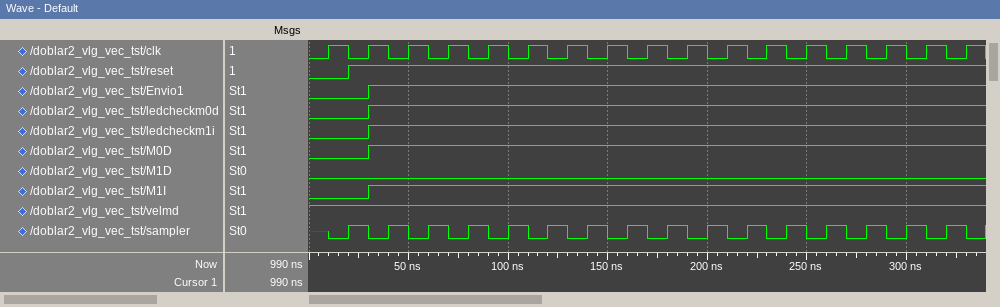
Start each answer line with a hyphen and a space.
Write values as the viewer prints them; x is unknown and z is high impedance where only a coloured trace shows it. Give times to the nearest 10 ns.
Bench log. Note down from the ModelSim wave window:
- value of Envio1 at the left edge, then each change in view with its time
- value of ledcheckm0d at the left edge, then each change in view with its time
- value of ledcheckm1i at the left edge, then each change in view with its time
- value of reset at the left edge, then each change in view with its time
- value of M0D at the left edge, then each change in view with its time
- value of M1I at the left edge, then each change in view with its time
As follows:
- 0, 1 at 30 ns
- 0, 1 at 30 ns
- 0, 1 at 30 ns
- 0, 1 at 20 ns
- 0, 1 at 30 ns
- 0, 1 at 30 ns
